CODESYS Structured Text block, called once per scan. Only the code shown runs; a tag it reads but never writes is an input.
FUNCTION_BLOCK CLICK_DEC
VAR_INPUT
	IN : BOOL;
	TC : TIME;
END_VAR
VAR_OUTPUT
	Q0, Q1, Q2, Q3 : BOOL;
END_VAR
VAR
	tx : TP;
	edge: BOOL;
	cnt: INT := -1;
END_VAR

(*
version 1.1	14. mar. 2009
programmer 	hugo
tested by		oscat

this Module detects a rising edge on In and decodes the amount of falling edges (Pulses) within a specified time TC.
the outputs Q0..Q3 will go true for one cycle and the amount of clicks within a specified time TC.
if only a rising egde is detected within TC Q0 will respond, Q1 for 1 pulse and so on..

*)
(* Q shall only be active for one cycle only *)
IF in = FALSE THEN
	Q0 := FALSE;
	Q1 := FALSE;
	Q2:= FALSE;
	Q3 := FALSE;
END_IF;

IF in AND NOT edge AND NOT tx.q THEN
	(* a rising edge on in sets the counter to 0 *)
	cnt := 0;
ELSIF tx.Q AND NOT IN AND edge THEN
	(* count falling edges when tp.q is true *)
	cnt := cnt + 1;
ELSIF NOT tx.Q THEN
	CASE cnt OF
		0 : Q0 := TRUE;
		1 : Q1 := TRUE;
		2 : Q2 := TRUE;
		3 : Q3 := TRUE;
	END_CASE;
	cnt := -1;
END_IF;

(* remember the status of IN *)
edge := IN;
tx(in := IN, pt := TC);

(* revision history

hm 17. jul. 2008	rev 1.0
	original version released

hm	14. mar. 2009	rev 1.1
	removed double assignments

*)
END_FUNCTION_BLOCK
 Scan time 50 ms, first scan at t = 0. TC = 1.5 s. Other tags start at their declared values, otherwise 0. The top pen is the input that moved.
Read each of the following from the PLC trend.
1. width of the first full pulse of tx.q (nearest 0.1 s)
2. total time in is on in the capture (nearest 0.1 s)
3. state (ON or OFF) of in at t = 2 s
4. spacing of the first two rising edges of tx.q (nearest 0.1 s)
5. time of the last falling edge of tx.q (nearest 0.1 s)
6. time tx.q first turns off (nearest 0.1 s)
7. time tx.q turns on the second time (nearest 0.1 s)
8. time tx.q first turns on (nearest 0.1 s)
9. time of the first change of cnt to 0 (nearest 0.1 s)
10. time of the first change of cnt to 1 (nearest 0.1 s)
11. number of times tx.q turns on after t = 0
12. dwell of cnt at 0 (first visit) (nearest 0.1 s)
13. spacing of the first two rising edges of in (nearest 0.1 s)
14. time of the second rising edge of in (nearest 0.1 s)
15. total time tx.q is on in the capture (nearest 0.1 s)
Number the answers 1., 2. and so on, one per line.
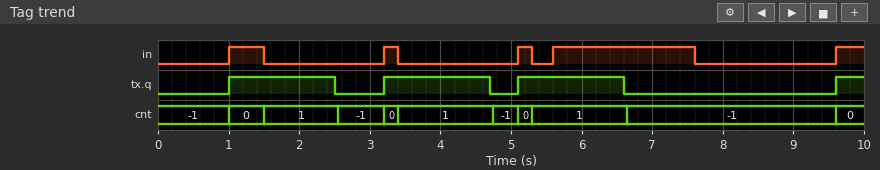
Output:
1. 1.5 s
2. 3.3 s
3. OFF
4. 2.2 s
5. 6.6 s
6. 2.5 s
7. 3.2 s
8. 1.0 s
9. 1.0 s
10. 1.5 s
11. 4
12. 0.5 s
13. 2.2 s
14. 3.2 s
15. 4.9 s
